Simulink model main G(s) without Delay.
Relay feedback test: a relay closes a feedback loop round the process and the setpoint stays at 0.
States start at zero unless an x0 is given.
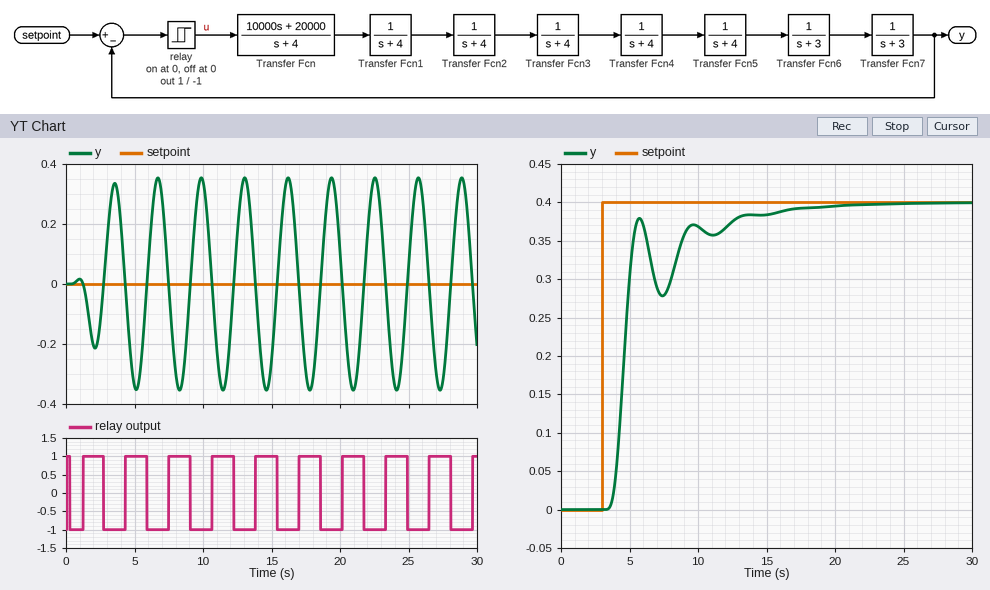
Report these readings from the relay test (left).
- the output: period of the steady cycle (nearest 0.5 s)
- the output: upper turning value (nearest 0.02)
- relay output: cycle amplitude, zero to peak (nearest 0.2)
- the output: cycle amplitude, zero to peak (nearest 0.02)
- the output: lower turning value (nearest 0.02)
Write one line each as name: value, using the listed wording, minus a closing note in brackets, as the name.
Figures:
the output: period of the steady cycle: 3.0 s
the output: upper turning value: 0.36
relay output: cycle amplitude, zero to peak: 1.0
the output: cycle amplitude, zero to peak: 0.36
the output: lower turning value: -0.36
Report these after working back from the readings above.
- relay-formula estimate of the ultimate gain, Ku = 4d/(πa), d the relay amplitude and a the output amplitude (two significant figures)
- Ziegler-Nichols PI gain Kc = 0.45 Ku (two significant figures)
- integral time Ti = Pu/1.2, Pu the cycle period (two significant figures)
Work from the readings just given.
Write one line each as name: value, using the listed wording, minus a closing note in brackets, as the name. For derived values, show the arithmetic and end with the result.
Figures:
relay-formula estimate of the ultimate gain, Ku = 4d/(πa), d the relay amplitude and a the output amplitude: 4 × 1 / (π × 0.36) = 3.5
Ziegler-Nichols PI gain Kc = 0.45 Ku: 0.45 × 3.5 = 1.6
integral time Ti = Pu/1.2, Pu the cycle period: 3 / 1.2 = 2.5 s
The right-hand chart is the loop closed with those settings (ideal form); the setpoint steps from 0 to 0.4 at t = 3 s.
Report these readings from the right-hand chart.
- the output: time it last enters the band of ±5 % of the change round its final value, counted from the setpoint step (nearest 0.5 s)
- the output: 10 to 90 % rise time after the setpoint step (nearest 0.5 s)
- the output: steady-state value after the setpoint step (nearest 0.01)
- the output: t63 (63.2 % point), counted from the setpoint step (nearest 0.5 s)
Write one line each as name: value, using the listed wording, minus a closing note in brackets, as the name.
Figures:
the output: time it last enters the band of ±5 % of the change round its final value, counted from the setpoint step: 10.0 s
the output: 10 to 90 % rise time after the setpoint step: 1.5 s
the output: steady-state value after the setpoint step: 0.40
the output: t63 (63.2 % point), counted from the setpoint step: 2.0 s
